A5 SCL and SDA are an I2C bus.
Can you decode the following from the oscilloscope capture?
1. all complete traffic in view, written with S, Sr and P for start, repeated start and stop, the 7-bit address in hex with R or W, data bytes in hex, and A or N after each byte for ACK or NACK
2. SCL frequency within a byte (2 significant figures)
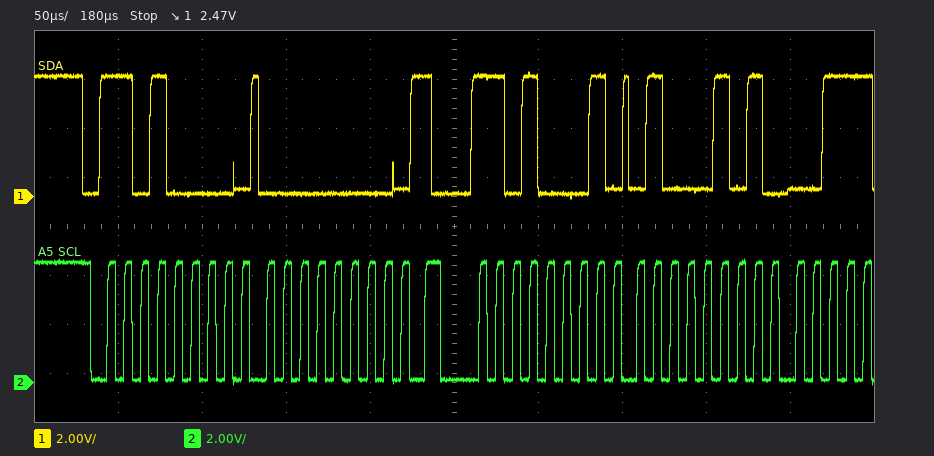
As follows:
S 68W A 00 A Sr 68R A 45 A
100 kHz
